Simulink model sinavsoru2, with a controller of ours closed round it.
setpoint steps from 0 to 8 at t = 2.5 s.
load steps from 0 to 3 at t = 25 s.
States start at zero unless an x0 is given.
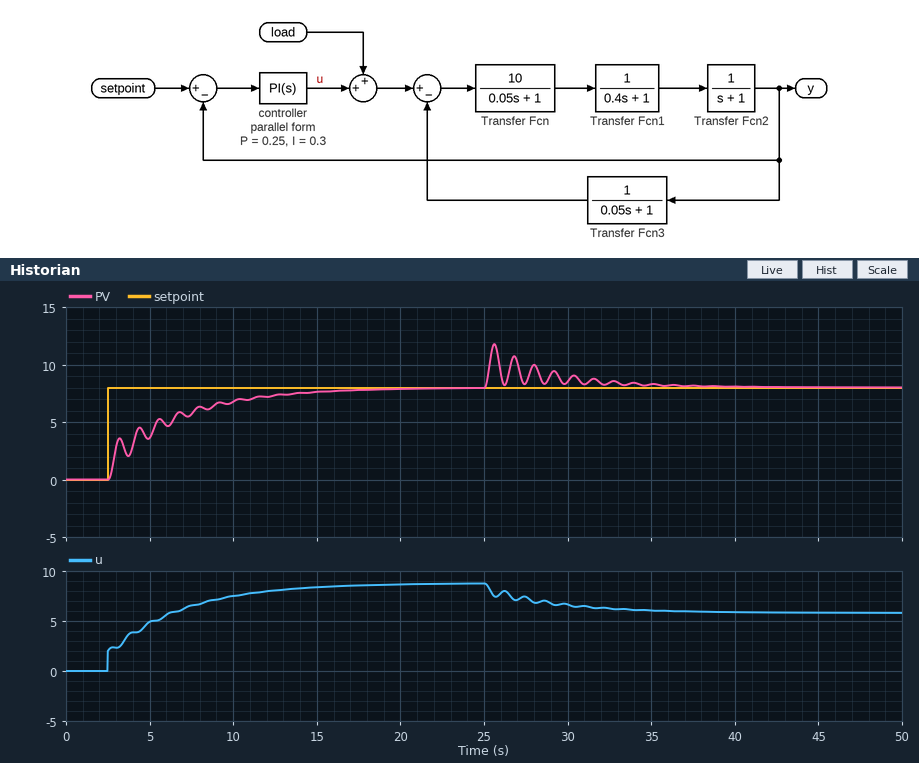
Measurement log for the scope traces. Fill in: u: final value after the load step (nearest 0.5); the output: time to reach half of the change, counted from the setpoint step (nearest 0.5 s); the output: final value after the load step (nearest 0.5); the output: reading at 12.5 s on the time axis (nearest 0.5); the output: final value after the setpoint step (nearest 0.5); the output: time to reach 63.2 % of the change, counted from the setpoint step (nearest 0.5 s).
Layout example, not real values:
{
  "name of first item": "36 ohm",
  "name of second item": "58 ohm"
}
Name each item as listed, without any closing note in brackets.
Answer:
{
  "u: final value after the load step": "6.0",
  "the output: time to reach half of the change, counted from the setpoint step": "1.5 s",
  "the output: final value after the load step": "8.0",
  "the output: reading at 12.5 s on the time axis": "7.5",
  "the output: final value after the setpoint step": "8.0",
  "the output: time to reach 63.2 % of the change, counted from the setpoint step": "3.0 s"
}
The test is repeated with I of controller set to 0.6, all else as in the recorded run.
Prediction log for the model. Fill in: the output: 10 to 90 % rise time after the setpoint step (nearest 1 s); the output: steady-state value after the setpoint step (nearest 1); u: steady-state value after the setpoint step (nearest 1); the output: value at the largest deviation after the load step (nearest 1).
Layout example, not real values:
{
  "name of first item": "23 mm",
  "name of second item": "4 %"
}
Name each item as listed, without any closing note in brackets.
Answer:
{
  "the output: 10 to 90 % rise time after the setpoint step": "3 s",
  "the output: steady-state value after the setpoint step": "8",
  "u: steady-state value after the setpoint step": "9",
  "the output: value at the largest deviation after the load step": "12"
}
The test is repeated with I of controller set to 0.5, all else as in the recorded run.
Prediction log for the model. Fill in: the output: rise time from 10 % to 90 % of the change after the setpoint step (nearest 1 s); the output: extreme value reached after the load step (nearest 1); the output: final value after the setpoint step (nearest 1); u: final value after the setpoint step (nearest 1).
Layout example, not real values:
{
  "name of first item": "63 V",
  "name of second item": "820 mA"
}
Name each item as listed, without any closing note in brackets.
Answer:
{
  "the output: rise time from 10 % to 90 % of the change after the setpoint step": "4 s",
  "the output: extreme value reached after the load step": "12",
  "the output: final value after the setpoint step": "8",
  "u: final value after the setpoint step": "9"
}
